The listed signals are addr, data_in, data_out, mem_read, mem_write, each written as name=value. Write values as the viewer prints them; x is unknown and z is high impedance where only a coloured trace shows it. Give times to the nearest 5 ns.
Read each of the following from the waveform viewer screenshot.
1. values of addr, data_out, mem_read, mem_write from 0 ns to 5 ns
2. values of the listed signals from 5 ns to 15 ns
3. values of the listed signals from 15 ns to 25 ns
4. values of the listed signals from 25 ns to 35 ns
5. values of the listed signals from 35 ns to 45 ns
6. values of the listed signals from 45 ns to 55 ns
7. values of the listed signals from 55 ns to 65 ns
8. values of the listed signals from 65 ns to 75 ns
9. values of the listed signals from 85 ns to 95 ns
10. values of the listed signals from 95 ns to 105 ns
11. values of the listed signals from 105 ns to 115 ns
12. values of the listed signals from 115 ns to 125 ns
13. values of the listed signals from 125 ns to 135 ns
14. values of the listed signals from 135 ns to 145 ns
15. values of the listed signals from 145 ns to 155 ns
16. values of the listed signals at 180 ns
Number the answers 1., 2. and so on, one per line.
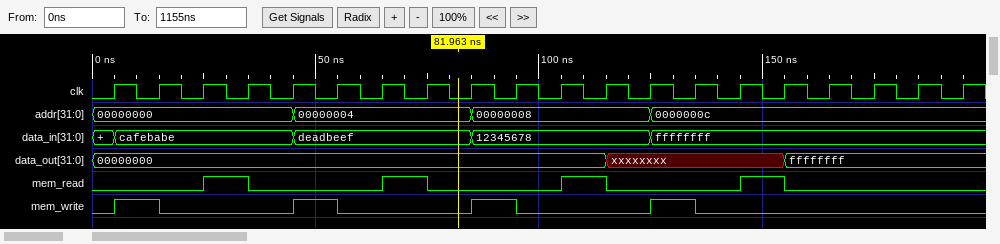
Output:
1. addr=00000000, data_out=00000000, mem_read=0, mem_write=0
2. addr=00000000, data_in=cafebabe, data_out=00000000, mem_read=0, mem_write=1
3. addr=00000000, data_in=cafebabe, data_out=00000000, mem_read=0, mem_write=0
4. addr=00000000, data_in=cafebabe, data_out=00000000, mem_read=1, mem_write=0
5. addr=00000000, data_in=cafebabe, data_out=00000000, mem_read=0, mem_write=0
6. addr=00000004, data_in=deadbeef, data_out=00000000, mem_read=0, mem_write=1
7. addr=00000004, data_in=deadbeef, data_out=00000000, mem_read=0, mem_write=0
8. addr=00000004, data_in=deadbeef, data_out=00000000, mem_read=1, mem_write=0
9. addr=00000008, data_in=12345678, data_out=00000000, mem_read=0, mem_write=1
10. addr=00000008, data_in=12345678, data_out=00000000, mem_read=0, mem_write=0
11. addr=00000008, data_in=12345678, data_out=00000000, mem_read=1, mem_write=0
12. addr=00000008, data_in=12345678, data_out=xxxxxxxx, mem_read=0, mem_write=0
13. addr=0000000c, data_in=ffffffff, data_out=xxxxxxxx, mem_read=0, mem_write=1
14. addr=0000000c, data_in=ffffffff, data_out=xxxxxxxx, mem_read=0, mem_write=0
15. addr=0000000c, data_in=ffffffff, data_out=xxxxxxxx, mem_read=1, mem_write=0
16. addr=0000000c, data_in=ffffffff, data_out=ffffffff, mem_read=0, mem_write=0
